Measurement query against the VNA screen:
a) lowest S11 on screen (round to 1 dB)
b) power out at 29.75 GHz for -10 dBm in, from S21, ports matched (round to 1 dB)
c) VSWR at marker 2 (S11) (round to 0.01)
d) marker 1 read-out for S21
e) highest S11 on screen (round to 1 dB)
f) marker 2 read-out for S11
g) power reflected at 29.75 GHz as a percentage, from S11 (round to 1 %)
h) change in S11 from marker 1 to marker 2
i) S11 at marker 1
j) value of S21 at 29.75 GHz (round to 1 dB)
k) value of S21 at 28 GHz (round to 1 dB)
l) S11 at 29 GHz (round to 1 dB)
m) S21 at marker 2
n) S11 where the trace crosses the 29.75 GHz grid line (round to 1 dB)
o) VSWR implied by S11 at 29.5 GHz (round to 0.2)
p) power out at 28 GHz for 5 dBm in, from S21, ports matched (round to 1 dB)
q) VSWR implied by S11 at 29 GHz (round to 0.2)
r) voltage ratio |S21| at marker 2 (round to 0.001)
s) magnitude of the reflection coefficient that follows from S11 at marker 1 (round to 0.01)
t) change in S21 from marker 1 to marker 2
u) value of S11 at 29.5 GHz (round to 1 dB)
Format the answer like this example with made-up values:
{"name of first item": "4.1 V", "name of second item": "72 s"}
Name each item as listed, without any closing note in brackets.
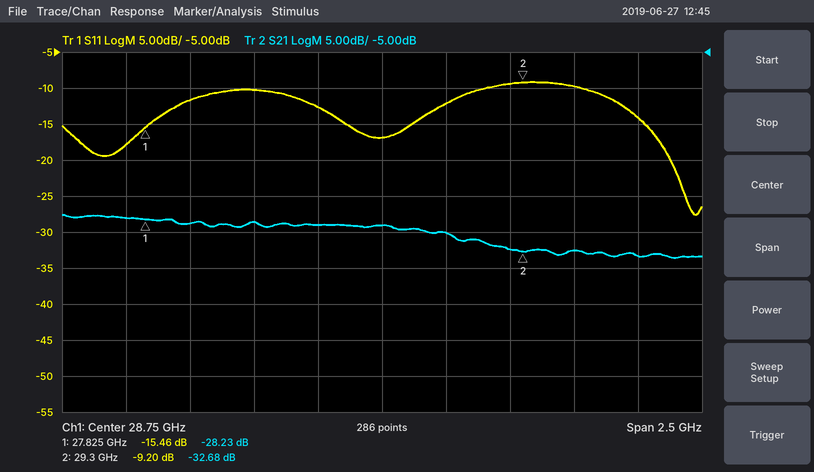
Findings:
{"lowest S11 on screen": "-28 dB", "power out at 29.75 GHz for -10 dBm in, from S21, ports matched": "-43 dBm", "VSWR at marker 2 (S11)": "2.06", "marker 1 read-out for S21": "-28.23 dB", "highest S11 on screen": "-9 dB", "marker 2 read-out for S11": "-9.20 dB", "power reflected at 29.75 GHz as a percentage, from S11": "4 %", "change in S11 from marker 1 to marker 2": "6.26 dB", "S11 at marker 1": "-15.46 dB", "value of S21 at 29.75 GHz": "-33 dB", "value of S21 at 28 GHz": "-29 dB", "S11 at 29 GHz": "-12 dB", "S21 at marker 2": "-32.68 dB", "S11 where the trace crosses the 29.75 GHz grid line": "-14 dB", "VSWR implied by S11 at 29.5 GHz": "2.0", "power out at 28 GHz for 5 dBm in, from S21, ports matched": "-24 dBm", "VSWR implied by S11 at 29 GHz": "1.6", "voltage ratio |S21| at marker 2": "0.023", "magnitude of the reflection coefficient that follows from S11 at marker 1": "0.17", "change in S21 from marker 1 to marker 2": "-4.45 dB", "value of S11 at 29.5 GHz": "-10 dB"}
